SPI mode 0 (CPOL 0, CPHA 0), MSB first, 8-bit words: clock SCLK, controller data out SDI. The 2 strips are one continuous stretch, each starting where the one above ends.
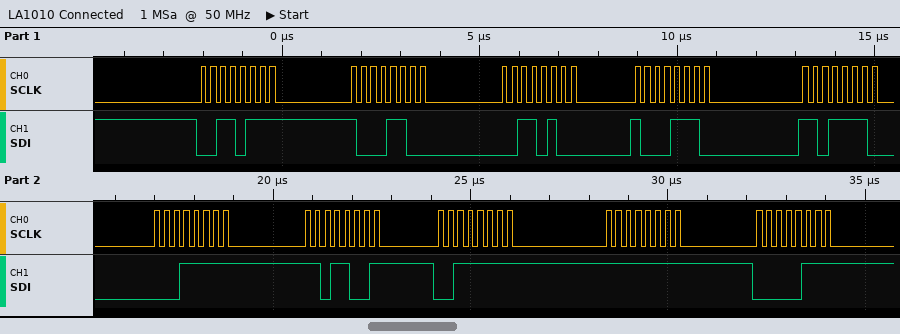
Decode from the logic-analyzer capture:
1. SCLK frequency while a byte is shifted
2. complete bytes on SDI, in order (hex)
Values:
4 MHz
37 8C 34 8E DE 1F D9 3F FF 07
